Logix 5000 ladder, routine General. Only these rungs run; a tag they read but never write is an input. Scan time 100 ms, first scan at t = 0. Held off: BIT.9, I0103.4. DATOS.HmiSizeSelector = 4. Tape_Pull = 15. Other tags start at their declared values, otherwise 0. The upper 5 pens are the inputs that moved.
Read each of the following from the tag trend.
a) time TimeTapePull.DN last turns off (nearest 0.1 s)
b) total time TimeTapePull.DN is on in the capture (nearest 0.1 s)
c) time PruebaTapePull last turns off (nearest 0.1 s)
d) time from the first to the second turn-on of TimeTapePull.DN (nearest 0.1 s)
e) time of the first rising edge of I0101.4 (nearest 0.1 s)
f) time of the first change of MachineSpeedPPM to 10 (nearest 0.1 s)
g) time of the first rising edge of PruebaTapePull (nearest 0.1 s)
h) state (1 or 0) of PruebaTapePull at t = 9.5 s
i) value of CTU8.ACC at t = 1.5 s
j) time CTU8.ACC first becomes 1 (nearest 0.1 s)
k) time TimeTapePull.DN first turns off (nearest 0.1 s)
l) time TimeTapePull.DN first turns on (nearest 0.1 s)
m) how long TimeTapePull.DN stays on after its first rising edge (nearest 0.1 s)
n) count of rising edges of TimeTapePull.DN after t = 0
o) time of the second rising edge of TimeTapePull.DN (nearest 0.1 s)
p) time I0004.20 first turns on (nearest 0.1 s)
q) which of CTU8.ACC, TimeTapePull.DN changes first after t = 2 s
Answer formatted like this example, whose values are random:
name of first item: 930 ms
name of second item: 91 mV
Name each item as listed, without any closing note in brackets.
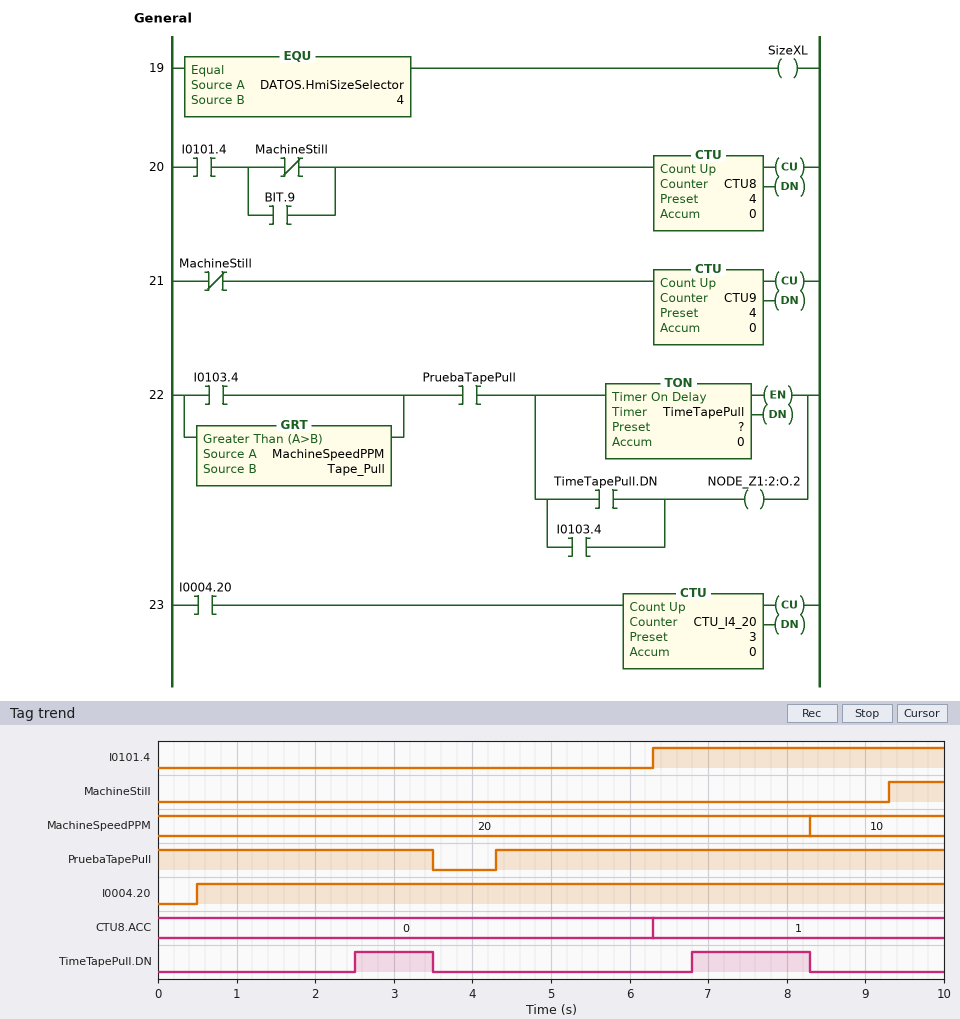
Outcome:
time TimeTapePull.DN last turns off: 8.3 s
total time TimeTapePull.DN is on in the capture: 2.5 s
time PruebaTapePull last turns off: 3.5 s
time from the first to the second turn-on of TimeTapePull.DN: 4.3 s
time of the first rising edge of I0101.4: 6.3 s
time of the first change of MachineSpeedPPM to 10: 8.3 s
time of the first rising edge of PruebaTapePull: 4.3 s
state (1 or 0) of PruebaTapePull at t = 9.5 s: 1
value of CTU8.ACC at t = 1.5 s: 0
time CTU8.ACC first becomes 1: 6.3 s
time TimeTapePull.DN first turns off: 3.5 s
time TimeTapePull.DN first turns on: 2.5 s
how long TimeTapePull.DN stays on after its first rising edge: 1.0 s
count of rising edges of TimeTapePull.DN after t = 0: 2
time of the second rising edge of TimeTapePull.DN: 6.8 s
time I0004.20 first turns on: 0.5 s
which of CTU8.ACC, TimeTapePull.DN changes first after t = 2 s: TimeTapePull.DN
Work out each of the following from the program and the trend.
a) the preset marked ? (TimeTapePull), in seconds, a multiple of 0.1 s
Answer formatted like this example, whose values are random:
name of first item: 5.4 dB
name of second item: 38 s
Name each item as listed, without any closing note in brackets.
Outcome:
the preset marked ? (TimeTapePull), in seconds, a multiple of 0.1 s: 2.5 s
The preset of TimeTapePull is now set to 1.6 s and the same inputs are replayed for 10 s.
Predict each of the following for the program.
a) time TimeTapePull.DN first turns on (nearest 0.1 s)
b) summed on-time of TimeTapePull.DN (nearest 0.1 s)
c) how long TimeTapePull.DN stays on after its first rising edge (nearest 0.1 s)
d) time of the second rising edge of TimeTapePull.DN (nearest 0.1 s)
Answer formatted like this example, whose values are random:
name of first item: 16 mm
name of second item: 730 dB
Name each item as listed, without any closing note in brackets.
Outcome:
time TimeTapePull.DN first turns on: 1.6 s
summed on-time of TimeTapePull.DN: 4.3 s
how long TimeTapePull.DN stays on after its first rising edge: 1.9 s
time of the second rising edge of TimeTapePull.DN: 5.9 s
